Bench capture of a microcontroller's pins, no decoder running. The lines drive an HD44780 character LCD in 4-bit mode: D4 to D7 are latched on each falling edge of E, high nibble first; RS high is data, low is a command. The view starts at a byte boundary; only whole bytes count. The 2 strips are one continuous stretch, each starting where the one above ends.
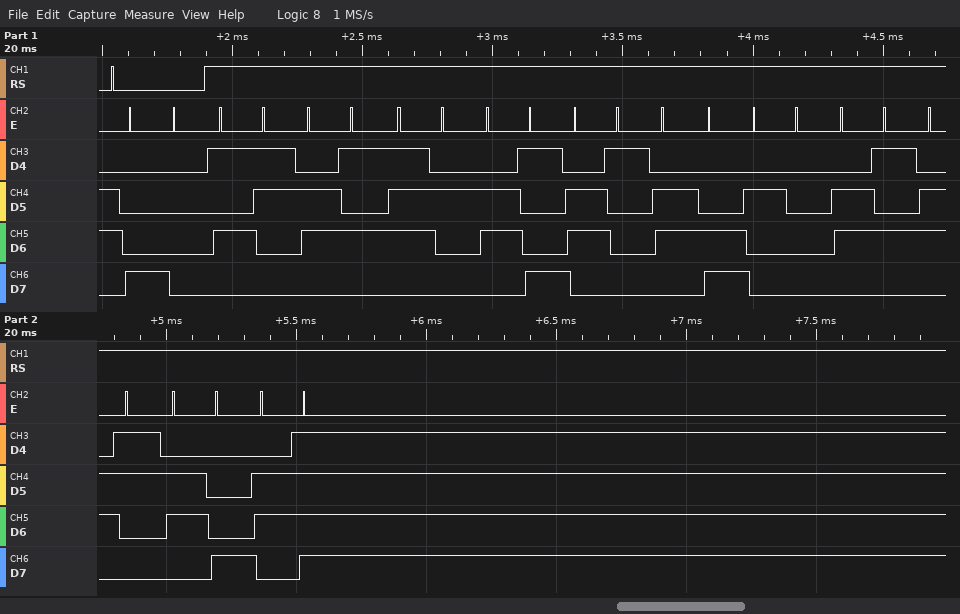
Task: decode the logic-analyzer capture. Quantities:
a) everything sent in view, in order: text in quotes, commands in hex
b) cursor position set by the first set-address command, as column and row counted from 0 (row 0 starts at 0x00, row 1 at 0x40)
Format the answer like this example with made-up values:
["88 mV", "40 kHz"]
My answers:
["0x80 \"Serial echo\"", "column 0, row 0"]
